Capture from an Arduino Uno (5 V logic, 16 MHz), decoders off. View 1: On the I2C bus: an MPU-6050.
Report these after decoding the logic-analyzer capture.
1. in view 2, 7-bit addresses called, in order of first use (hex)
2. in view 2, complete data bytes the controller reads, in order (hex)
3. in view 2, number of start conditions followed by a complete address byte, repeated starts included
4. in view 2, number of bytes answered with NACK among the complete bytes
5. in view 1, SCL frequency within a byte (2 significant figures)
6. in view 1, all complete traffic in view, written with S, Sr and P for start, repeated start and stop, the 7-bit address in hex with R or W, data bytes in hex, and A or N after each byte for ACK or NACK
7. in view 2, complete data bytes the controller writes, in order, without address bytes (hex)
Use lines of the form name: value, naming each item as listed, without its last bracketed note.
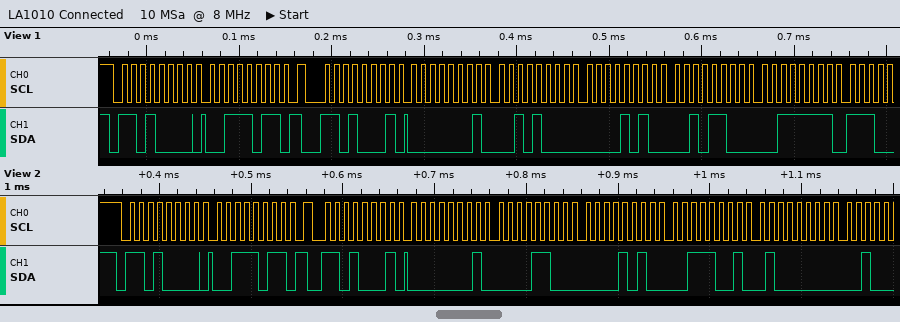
in view 2, 7-bit addresses called, in order of first use: 0x68
in view 2, complete data bytes the controller reads, in order: 01 0C 0A 39 40
in view 2, number of start conditions followed by a complete address byte, repeated starts included: 2
in view 2, number of bytes answered with NACK among the complete bytes: 0
in view 1, SCL frequency within a byte: 100 kHz
in view 1, all complete traffic in view, written with S, Sr and P for start, repeated start and stop, the 7-bit address in hex with R or W, data bytes in hex, and A or N after each byte for ACK or NACK: S 68W A 3B A Sr 68R A 01 A 28 A 0A A 2C A 3F A
in view 2, complete data bytes the controller writes, in order, without address bytes: 3B
